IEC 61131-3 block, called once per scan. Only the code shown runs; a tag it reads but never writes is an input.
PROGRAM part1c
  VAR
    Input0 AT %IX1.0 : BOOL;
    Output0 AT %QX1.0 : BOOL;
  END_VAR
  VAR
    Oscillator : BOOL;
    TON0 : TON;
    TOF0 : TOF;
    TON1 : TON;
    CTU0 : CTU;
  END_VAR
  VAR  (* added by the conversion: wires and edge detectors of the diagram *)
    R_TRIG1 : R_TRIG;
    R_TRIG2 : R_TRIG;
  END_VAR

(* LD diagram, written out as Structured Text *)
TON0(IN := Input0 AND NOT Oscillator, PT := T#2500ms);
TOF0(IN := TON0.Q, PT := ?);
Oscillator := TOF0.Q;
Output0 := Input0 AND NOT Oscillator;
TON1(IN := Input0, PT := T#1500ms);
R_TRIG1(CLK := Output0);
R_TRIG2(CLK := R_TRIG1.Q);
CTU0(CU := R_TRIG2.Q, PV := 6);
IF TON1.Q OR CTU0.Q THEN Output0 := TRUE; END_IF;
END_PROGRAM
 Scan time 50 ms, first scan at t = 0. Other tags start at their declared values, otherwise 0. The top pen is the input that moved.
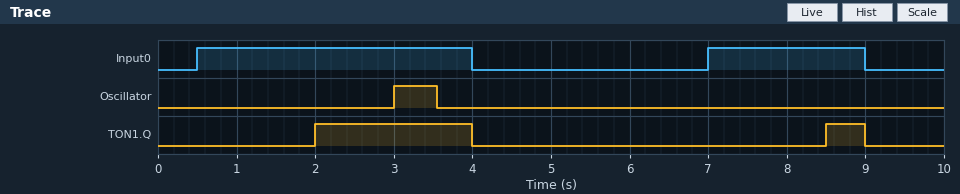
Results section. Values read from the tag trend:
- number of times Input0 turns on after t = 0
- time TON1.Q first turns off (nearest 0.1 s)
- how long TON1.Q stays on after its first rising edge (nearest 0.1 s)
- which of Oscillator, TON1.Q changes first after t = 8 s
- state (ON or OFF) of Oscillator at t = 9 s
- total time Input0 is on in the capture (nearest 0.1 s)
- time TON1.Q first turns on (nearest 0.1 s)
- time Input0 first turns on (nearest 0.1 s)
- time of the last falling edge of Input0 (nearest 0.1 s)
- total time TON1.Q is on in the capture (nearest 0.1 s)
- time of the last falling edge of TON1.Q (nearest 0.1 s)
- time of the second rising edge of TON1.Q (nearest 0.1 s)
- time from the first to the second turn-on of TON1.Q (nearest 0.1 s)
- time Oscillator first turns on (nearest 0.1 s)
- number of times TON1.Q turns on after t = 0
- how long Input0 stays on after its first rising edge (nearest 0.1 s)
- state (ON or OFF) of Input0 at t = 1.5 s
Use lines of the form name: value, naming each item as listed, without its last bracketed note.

number of times Input0 turns on after t = 0: 2
time TON1.Q first turns off: 4.0 s
how long TON1.Q stays on after its first rising edge: 2.0 s
which of Oscillator, TON1.Q changes first after t = 8 s: TON1.Q
state (ON or OFF) of Oscillator at t = 9 s: OFF
total time Input0 is on in the capture: 5.5 s
time TON1.Q first turns on: 2.0 s
time Input0 first turns on: 0.5 s
time of the last falling edge of Input0: 9.0 s
total time TON1.Q is on in the capture: 2.5 s
time of the last falling edge of TON1.Q: 9.0 s
time of the second rising edge of TON1.Q: 8.5 s
time from the first to the second turn-on of TON1.Q: 6.5 s
time Oscillator first turns on: 3.0 s
number of times TON1.Q turns on after t = 0: 2
how long Input0 stays on after its first rising edge: 3.5 s
state (ON or OFF) of Input0 at t = 1.5 s: ON
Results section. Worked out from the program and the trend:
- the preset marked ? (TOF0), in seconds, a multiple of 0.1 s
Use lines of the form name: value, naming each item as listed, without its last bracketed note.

the preset marked ? (TOF0), in seconds, a multiple of 0.1 s: 0.5 s
